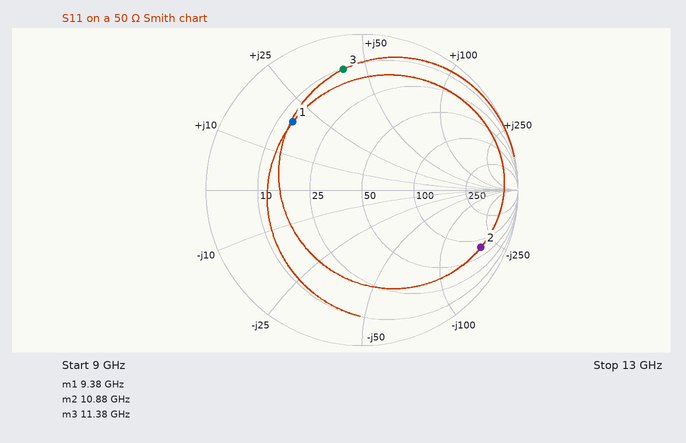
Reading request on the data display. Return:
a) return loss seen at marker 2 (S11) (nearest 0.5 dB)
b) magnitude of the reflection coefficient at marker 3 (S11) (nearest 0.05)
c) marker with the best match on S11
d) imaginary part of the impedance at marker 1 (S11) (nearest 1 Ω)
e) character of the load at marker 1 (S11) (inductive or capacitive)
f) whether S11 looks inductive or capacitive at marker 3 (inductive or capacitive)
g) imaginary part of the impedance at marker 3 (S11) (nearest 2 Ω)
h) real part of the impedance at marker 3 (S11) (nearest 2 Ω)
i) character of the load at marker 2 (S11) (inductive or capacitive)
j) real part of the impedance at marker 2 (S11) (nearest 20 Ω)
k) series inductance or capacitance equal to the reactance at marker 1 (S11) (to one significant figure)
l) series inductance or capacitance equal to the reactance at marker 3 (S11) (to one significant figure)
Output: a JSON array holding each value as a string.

["1.5 dB", "0.80", "marker 1", "+19 Ω", "inductive", "inductive", "+42 Ω", "10 Ω", "capacitive", "80 Ω", "300 pH", "600 pH"]
